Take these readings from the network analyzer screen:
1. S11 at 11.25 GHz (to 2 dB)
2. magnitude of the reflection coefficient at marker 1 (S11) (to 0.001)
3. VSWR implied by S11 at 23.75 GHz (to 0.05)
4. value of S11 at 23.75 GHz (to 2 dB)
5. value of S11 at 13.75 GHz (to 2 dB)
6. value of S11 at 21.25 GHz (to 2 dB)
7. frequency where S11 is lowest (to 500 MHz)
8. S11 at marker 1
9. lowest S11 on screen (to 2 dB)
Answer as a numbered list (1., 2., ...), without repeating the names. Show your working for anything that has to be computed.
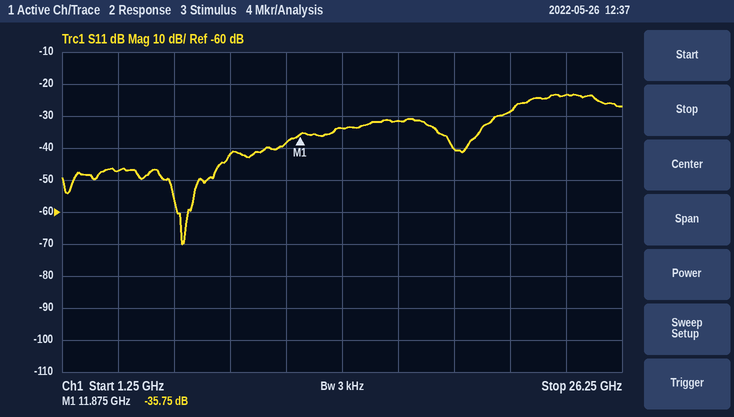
1. -38 dB
2. 10^(-35.75/20) ≈ 0.016
3. |Γ| = 10^(-24/20) = 0.0631; VSWR = (1 + 0.0631)/(1 − 0.0631) ≈ 1.13, so 1.15 to the nearest 0.05
4. -24 dB
5. -34 dB
6. -28 dB
7. 6.5 GHz
8. -35.75 dB
9. -70 dB
